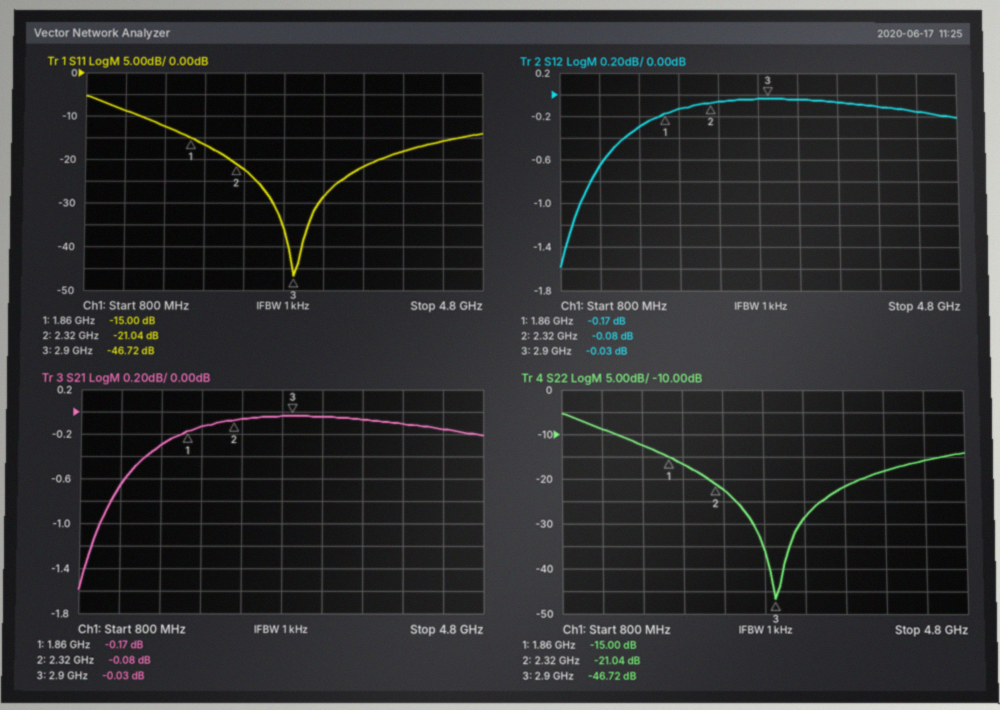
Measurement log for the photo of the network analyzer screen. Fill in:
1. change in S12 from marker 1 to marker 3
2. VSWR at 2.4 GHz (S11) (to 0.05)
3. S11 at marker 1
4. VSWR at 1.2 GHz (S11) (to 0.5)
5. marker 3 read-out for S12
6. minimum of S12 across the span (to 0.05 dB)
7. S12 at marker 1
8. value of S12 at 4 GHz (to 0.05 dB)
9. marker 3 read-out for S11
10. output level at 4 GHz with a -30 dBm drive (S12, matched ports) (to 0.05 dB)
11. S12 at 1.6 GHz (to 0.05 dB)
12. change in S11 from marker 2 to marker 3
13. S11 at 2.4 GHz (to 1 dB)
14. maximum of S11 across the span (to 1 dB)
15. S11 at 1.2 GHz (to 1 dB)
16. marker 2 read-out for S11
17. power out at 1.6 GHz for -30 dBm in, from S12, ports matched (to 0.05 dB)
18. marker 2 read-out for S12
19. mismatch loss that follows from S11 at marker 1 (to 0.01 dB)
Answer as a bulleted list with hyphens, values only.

- 0.14 dB
- 1.15
- -15.00 dB
- 2.0
- -0.03 dB
- -1.60 dB
- -0.17 dB
- -0.10 dB
- -46.72 dB
- -30.10 dBm
- -0.30 dB
- -25.68 dB
- -22 dB
- -5 dB
- -9 dB
- -21.04 dB
- -30.30 dBm
- -0.08 dB
- 0.14 dB
